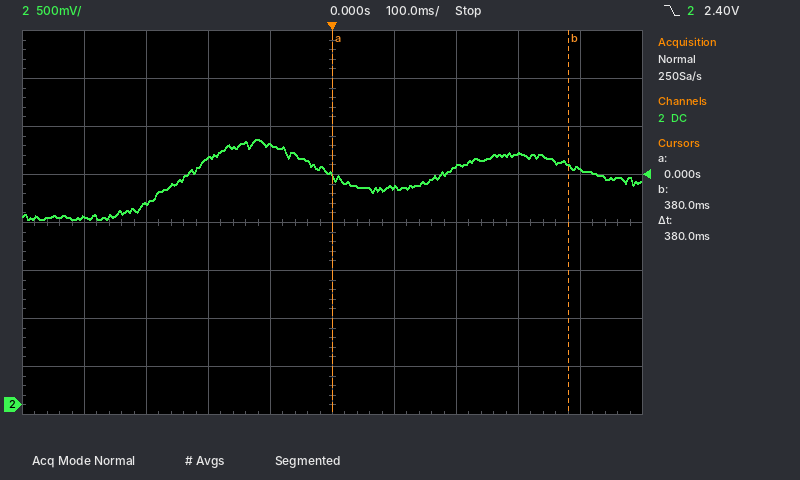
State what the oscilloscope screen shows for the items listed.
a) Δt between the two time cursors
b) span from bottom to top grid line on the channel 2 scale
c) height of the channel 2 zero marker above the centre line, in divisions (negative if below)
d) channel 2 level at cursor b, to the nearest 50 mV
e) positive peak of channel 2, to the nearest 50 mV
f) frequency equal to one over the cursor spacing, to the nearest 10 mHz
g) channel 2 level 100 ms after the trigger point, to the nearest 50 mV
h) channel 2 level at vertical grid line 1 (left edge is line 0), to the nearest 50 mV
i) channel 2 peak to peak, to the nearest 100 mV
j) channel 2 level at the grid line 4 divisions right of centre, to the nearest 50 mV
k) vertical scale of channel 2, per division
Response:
380 ms
4 V
-3.8 div
2.50 V
2.75 V
2.63 Hz
2.25 V
1.95 V
800 mV
2.45 V
500 mV
